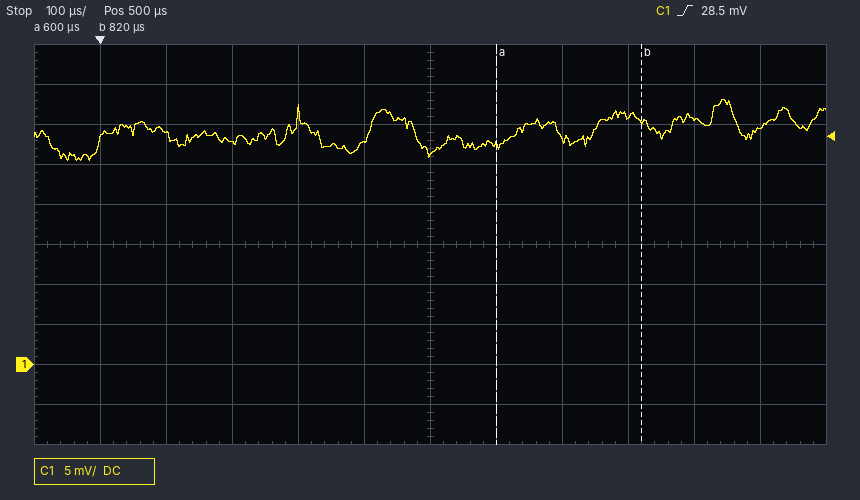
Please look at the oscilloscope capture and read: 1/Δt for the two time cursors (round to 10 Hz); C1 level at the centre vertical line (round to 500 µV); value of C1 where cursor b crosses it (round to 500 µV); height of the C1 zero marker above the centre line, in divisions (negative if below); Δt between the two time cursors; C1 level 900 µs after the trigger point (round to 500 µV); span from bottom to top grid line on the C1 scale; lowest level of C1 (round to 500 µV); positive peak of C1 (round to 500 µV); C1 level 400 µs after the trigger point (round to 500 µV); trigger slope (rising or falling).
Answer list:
4.55 kHz
26.5 mV
30.5 mV
-3.0 div
220 µs
30.5 mV
50 mV
25.5 mV
33.0 mV
28.0 mV
rising
